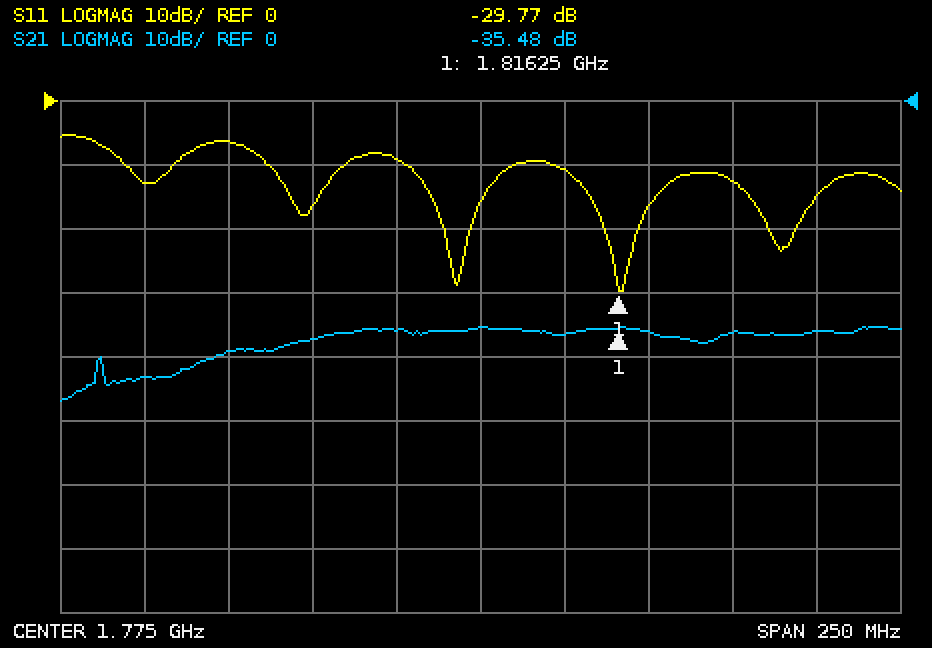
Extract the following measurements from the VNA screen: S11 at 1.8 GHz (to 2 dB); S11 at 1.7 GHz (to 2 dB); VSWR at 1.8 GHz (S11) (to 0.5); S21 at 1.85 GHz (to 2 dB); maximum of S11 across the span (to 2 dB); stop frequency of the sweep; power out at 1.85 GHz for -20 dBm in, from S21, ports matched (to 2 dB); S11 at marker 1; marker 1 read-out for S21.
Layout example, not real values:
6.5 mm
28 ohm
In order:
-10 dB
-6 dB
2.0
-36 dB
-6 dB
1.9 GHz
-56 dBm
-29.77 dB
-35.48 dB
